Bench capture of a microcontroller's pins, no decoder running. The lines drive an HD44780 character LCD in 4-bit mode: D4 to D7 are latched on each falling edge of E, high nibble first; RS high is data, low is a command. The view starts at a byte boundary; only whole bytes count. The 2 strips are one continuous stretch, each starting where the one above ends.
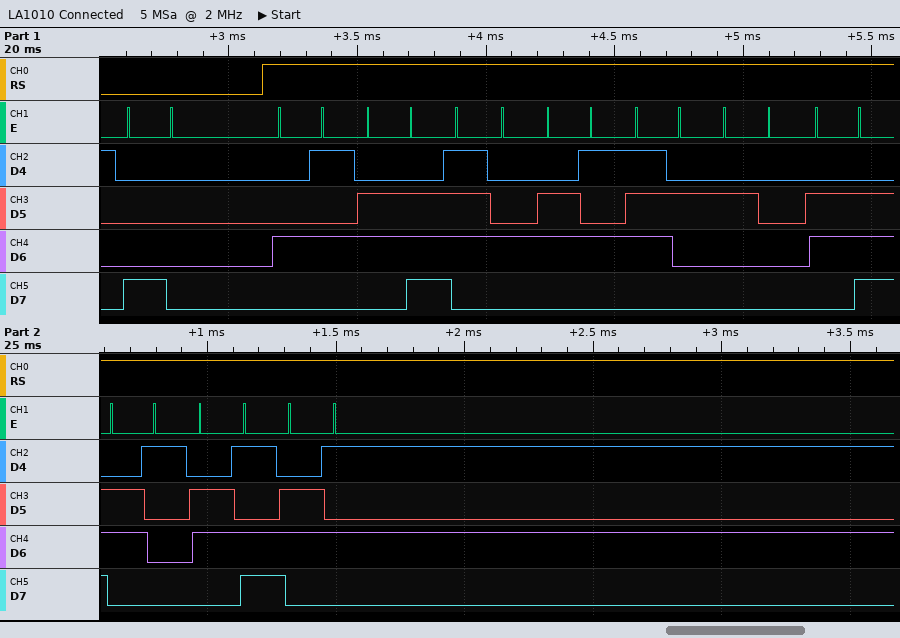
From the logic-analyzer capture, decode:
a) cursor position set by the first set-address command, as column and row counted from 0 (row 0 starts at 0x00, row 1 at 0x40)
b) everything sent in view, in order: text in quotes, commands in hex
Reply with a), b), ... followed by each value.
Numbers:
a) column 0, row 0
b) 0x80 "Enter name"
